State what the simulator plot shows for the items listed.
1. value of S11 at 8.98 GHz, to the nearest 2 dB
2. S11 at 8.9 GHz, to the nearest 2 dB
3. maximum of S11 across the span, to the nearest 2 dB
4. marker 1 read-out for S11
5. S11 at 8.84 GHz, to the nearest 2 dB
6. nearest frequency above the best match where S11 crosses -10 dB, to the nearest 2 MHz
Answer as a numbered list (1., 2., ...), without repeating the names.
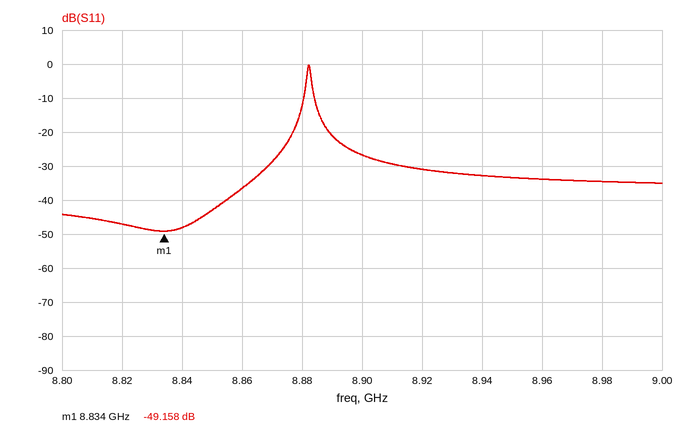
1. -34 dB
2. -26 dB
3. 0 dB
4. -49.158 dB
5. -48 dB
6. 8.880 GHz
